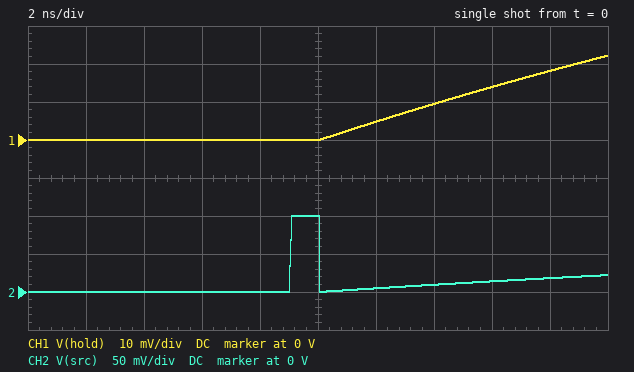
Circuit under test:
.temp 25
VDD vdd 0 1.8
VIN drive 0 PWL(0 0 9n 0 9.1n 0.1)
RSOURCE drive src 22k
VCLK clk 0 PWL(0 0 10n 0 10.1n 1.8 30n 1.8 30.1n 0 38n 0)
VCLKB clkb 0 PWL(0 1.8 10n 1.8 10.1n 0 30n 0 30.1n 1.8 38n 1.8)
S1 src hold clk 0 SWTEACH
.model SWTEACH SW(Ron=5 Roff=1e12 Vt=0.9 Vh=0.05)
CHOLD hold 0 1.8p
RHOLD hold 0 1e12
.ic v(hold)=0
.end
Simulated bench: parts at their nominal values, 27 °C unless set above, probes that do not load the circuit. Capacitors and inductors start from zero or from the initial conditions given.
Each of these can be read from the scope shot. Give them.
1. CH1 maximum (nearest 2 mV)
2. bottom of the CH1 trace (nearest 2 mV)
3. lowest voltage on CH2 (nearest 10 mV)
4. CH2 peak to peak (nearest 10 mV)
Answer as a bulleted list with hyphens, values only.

- 22 mV
- 0 V
- 0 V
- 100 mV
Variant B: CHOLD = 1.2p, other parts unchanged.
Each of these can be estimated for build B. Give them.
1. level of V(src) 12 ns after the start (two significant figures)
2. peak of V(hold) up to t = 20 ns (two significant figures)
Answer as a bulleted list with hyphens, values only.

- 7.1 mV
- 31 mV
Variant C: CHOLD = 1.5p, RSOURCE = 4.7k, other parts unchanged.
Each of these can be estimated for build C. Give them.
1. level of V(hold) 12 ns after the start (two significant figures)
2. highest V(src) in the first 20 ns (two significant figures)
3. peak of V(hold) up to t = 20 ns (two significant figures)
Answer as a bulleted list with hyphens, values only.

- 24 mV
- 100 mV
- 76 mV
